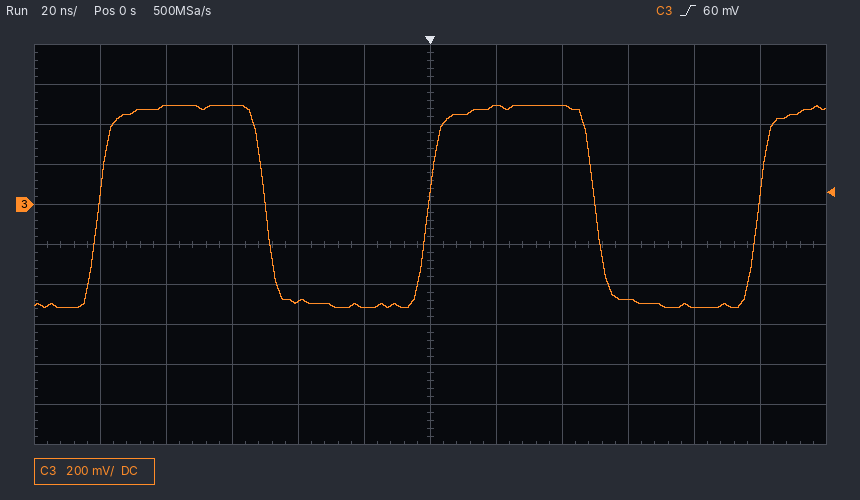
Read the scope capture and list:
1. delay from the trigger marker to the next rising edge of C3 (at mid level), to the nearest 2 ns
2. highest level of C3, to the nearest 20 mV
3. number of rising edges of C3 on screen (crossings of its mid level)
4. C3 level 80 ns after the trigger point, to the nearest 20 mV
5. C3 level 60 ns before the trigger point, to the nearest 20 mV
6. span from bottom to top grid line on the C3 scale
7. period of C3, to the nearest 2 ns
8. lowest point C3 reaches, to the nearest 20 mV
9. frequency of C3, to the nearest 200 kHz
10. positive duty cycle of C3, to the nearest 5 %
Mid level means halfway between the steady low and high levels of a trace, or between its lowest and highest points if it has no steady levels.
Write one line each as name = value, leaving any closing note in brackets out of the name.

delay from the trigger marker to the next rising edge of C3 (at mid level), to the nearest 2 ns = 100 ns
highest level of C3, to the nearest 20 mV = 500 mV
number of rising edges of C3 on screen = 3
C3 level 80 ns after the trigger point, to the nearest 20 mV = -520 mV
C3 level 60 ns before the trigger point, to the nearest 20 mV = 500 mV
span from bottom to top grid line on the C3 scale = 2 V
period of C3, to the nearest 2 ns = 100 ns
lowest point C3 reaches, to the nearest 20 mV = -520 mV
frequency of C3, to the nearest 200 kHz = 10.0 MHz
positive duty cycle of C3, to the nearest 5 % = 50 %
